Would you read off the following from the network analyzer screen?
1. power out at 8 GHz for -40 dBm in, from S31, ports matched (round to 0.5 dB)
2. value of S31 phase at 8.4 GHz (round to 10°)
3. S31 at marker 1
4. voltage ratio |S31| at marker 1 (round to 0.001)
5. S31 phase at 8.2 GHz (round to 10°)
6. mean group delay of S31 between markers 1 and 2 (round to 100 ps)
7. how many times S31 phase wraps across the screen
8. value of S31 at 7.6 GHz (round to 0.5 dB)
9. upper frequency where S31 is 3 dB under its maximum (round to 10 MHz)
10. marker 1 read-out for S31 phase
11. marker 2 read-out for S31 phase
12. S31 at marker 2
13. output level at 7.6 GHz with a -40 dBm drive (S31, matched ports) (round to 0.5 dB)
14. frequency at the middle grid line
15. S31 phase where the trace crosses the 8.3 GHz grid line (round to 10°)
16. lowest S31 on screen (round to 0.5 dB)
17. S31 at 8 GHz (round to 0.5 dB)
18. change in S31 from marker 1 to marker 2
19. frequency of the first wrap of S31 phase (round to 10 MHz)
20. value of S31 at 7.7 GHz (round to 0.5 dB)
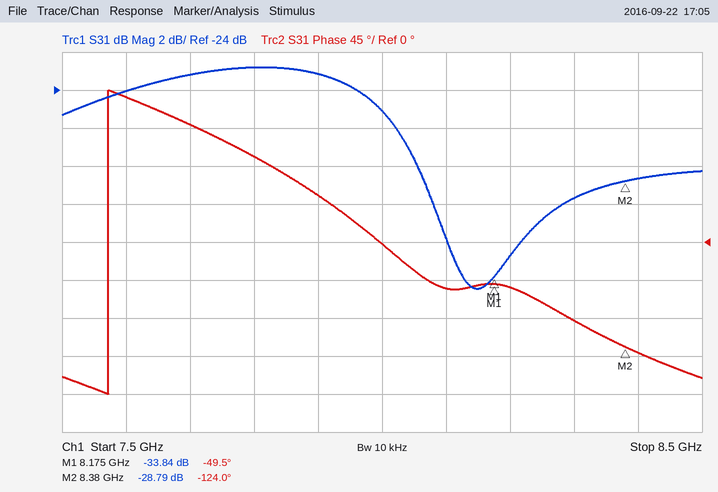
-65.0 dBm
-130°
-33.84 dB
0.020
-50°
1.0 ns
1
-24.0 dB
8.02 GHz
-49.5°
-124.0°
-28.79 dB
-64.0 dBm
8 GHz
-90°
-34.5 dB
-25.0 dB
5.05 dB
7.57 GHz
-23.0 dB
